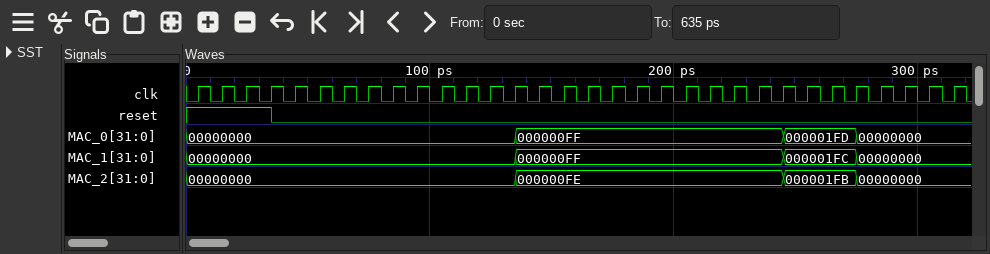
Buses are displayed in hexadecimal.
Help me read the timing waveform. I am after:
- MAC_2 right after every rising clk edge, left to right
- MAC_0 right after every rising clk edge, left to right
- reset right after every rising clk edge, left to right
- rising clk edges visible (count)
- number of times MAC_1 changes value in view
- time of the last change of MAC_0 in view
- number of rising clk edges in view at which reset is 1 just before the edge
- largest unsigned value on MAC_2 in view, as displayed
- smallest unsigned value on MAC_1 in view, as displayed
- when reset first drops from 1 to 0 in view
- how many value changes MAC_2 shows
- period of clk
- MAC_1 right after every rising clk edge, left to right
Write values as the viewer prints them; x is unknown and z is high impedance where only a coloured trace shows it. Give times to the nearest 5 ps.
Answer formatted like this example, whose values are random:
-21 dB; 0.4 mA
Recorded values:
00000000, 00000000, 00000000, 00000000, 00000000, 00000000, 00000000, 00000000, 00000000, 00000000, 00000000, 00000000, 00000000, 000000FE, 000000FE, 000000FE, 000000FE, 000000FE, 000000FE, 000000FE, 000000FE, 000000FE, 000000FE, 000000FE, 000001FB, 000001FB, 000001FB, 00000000, 00000000, 00000000, 00000000, 00000000; 00000000, 00000000, 00000000, 00000000, 00000000, 00000000, 00000000, 00000000, 00000000, 00000000, 00000000, 00000000, 00000000, 000000FF, 000000FF, 000000FF, 000000FF, 000000FF, 000000FF, 000000FF, 000000FF, 000000FF, 000000FF, 000000FF, 000001FD, 000001FD, 000001FD, 00000000, 00000000, 00000000, 00000000, 00000000; 1 1 1 0 0 0 0 0 0 0 0 0 0 0 0 0 0 0 0 0 0 0 0 0 0 0 0 0 0 0 0 0; 32; 3; 275 ps; 4; 000001FB; 00000000; 35 ps; 3; 10 ps; 00000000, 00000000, 00000000, 00000000, 00000000, 00000000, 00000000, 00000000, 00000000, 00000000, 00000000, 00000000, 00000000, 000000FF, 000000FF, 000000FF, 000000FF, 000000FF, 000000FF, 000000FF, 000000FF, 000000FF, 000000FF, 000000FF, 000001FC, 000001FC, 000001FC, 00000000, 00000000, 00000000, 00000000, 00000000
